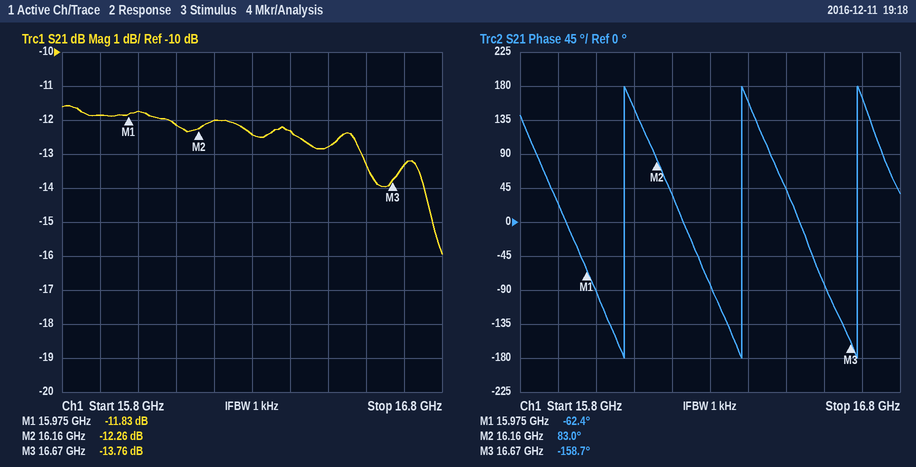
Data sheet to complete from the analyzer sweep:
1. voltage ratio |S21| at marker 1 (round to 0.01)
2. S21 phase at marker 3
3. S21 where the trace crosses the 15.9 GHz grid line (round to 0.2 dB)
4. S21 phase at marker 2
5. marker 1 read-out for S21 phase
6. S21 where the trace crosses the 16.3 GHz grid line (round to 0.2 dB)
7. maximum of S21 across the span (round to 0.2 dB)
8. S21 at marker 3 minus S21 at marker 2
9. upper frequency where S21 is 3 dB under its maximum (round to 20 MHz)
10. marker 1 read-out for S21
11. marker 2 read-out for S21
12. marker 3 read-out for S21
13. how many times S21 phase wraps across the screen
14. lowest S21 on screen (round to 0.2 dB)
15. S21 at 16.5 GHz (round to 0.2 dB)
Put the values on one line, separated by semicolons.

0.26; -158.7°; -11.8 dB; 83.0°; -62.4°; -12.4 dB; -11.6 dB; -1.50 dB; 16.76 GHz; -11.83 dB; -12.26 dB; -13.76 dB; 3; -16.0 dB; -12.8 dB
